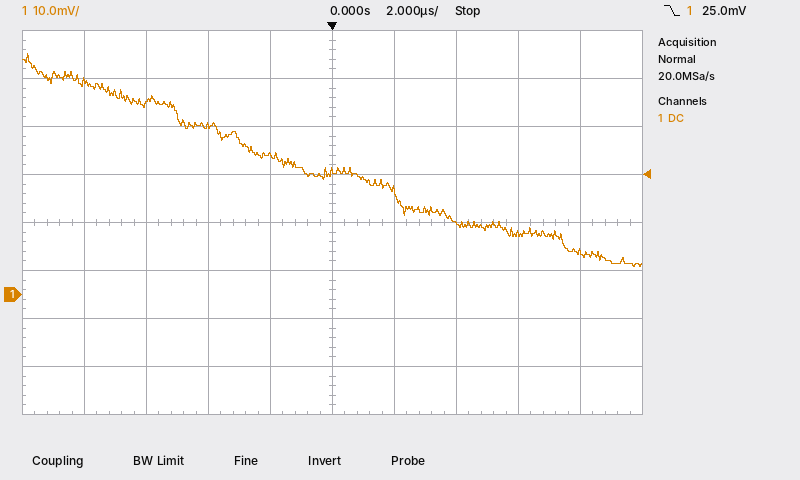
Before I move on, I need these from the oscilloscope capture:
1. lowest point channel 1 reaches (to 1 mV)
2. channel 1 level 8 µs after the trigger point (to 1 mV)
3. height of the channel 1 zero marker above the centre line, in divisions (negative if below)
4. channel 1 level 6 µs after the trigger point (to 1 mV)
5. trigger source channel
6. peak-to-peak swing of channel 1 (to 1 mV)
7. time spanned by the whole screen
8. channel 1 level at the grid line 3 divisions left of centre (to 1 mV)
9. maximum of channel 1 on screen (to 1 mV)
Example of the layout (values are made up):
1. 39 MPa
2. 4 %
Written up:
1. 6 mV
2. 9 mV
3. -1.5 div
4. 13 mV
5. channel 1
6. 44 mV
7. 20 µs
8. 40 mV
9. 50 mV
